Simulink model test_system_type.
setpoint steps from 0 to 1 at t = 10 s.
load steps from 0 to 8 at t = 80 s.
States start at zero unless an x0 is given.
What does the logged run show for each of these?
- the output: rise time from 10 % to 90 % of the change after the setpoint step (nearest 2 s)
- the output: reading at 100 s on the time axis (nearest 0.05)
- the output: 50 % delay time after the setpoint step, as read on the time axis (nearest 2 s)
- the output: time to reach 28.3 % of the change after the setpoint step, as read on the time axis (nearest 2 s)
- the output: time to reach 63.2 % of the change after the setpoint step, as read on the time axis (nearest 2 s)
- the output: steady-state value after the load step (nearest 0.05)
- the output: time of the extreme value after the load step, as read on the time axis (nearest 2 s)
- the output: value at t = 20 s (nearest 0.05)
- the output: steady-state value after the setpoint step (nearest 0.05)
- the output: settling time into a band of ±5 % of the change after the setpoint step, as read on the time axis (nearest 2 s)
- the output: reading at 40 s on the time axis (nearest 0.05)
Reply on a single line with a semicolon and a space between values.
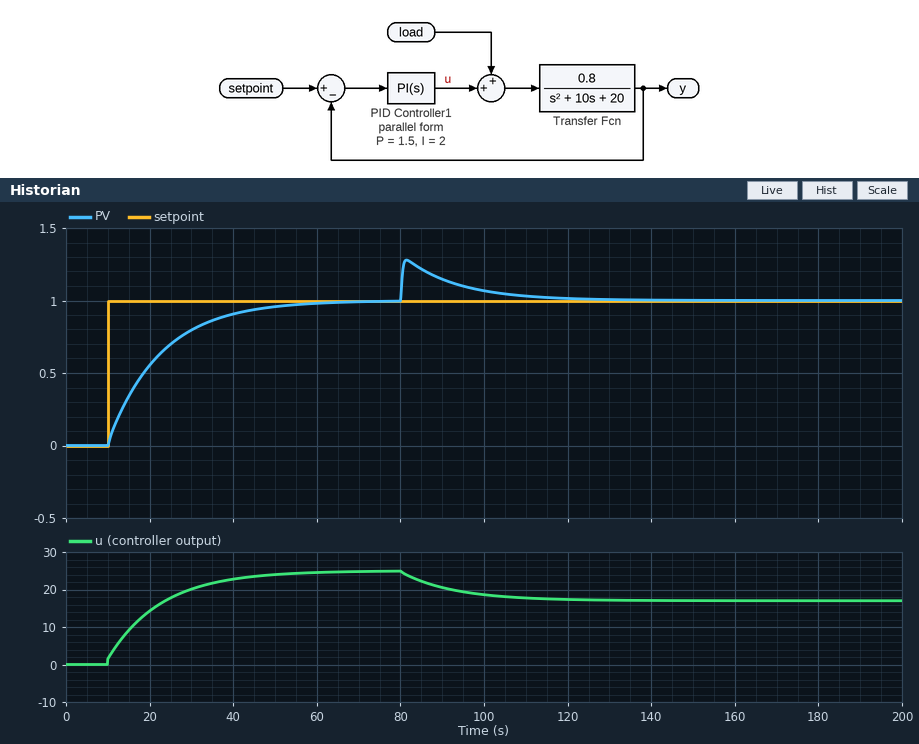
28 s; 1.05; 18 s; 14 s; 22 s; 1.00; 82 s; 0.55; 1.00; 48 s; 0.90
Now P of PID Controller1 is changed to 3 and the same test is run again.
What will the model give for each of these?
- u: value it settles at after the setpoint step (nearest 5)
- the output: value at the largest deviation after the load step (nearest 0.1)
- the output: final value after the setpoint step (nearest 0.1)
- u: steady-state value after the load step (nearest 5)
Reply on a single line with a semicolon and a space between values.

25; 1.3; 1.0; 15
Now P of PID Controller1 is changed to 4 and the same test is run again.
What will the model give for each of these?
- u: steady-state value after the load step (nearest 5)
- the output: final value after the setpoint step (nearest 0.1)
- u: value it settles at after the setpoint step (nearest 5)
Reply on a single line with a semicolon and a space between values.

15; 1.0; 25
